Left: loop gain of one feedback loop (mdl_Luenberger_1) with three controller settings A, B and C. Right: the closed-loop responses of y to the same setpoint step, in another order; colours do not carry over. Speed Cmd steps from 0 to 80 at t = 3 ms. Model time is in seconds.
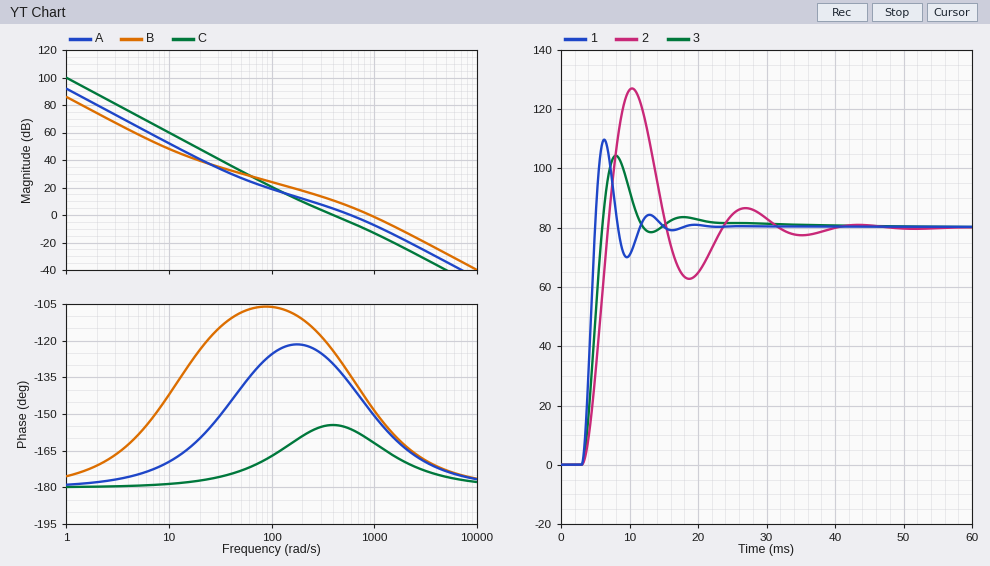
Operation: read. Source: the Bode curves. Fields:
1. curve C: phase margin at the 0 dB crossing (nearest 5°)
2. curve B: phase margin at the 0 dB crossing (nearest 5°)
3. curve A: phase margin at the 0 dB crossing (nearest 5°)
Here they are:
25°
35°
40°
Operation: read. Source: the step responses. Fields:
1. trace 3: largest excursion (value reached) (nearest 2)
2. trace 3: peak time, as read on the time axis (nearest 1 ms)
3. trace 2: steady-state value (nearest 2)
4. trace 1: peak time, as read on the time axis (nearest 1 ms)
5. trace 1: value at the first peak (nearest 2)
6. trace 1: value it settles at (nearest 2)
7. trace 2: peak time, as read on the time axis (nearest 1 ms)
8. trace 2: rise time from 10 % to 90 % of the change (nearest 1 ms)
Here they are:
104
8 ms
80
6 ms
110
80
10 ms
3 ms
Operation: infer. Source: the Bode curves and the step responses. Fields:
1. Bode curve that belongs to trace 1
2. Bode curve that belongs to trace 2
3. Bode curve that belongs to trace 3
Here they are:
B
C
A
